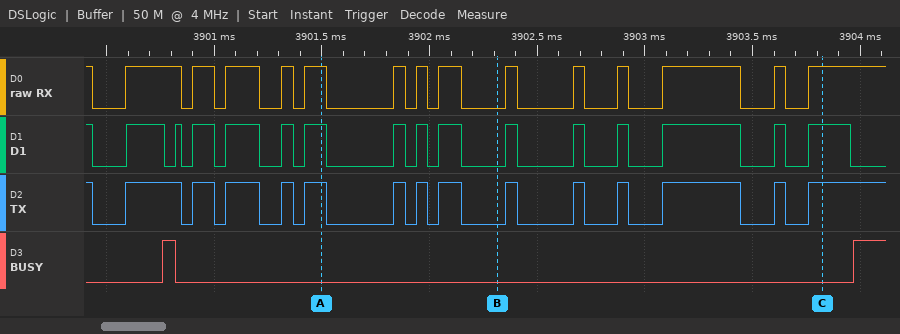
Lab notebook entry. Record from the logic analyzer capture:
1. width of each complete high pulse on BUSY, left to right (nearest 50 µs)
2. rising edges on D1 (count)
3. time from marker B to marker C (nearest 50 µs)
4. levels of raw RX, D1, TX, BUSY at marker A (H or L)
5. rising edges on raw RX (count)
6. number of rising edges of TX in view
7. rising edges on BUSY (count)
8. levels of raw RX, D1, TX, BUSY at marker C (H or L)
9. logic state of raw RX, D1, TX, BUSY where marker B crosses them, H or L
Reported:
50 µs
15
1500 µs
raw RX=H, D1=H, TX=H, BUSY=L
14
14
2
raw RX=H, D1=H, TX=H, BUSY=L
raw RX=L, D1=L, TX=L, BUSY=L
